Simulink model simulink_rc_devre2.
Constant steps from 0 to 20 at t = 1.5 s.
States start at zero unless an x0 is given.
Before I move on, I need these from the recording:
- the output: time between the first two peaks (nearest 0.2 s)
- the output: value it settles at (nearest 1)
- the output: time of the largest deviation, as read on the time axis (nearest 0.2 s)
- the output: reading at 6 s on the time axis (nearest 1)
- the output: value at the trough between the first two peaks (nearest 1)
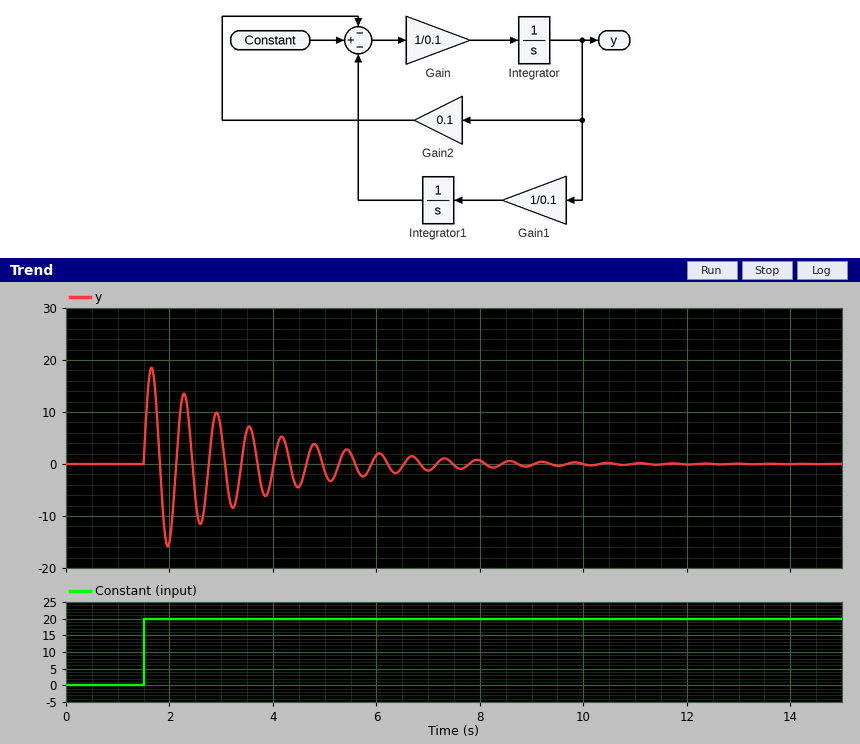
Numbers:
0.6 s
0
1.6 s
2
-16
